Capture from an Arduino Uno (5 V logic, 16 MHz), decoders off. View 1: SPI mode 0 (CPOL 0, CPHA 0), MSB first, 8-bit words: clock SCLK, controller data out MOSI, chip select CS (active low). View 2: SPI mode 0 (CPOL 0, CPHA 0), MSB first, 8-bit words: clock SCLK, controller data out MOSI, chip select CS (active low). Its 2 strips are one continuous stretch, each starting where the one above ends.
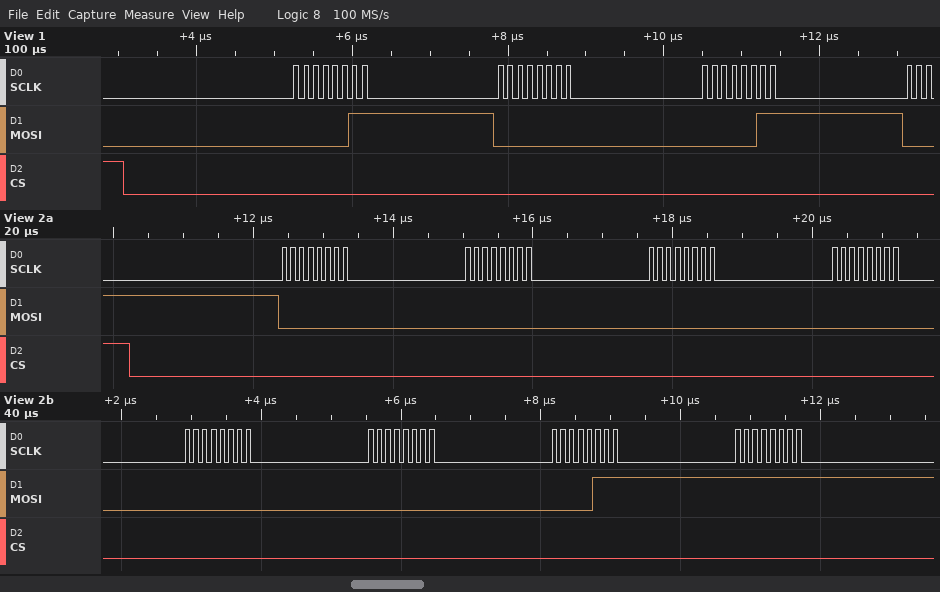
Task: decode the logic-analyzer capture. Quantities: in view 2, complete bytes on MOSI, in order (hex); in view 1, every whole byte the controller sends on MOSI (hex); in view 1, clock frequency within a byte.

00 00 00 00 00 00 07 FF
03 00 03
8 MHz
